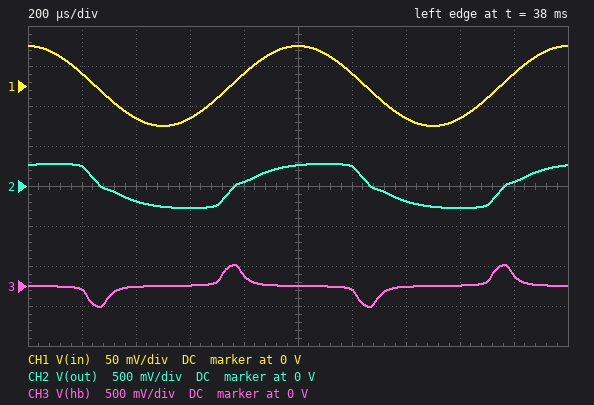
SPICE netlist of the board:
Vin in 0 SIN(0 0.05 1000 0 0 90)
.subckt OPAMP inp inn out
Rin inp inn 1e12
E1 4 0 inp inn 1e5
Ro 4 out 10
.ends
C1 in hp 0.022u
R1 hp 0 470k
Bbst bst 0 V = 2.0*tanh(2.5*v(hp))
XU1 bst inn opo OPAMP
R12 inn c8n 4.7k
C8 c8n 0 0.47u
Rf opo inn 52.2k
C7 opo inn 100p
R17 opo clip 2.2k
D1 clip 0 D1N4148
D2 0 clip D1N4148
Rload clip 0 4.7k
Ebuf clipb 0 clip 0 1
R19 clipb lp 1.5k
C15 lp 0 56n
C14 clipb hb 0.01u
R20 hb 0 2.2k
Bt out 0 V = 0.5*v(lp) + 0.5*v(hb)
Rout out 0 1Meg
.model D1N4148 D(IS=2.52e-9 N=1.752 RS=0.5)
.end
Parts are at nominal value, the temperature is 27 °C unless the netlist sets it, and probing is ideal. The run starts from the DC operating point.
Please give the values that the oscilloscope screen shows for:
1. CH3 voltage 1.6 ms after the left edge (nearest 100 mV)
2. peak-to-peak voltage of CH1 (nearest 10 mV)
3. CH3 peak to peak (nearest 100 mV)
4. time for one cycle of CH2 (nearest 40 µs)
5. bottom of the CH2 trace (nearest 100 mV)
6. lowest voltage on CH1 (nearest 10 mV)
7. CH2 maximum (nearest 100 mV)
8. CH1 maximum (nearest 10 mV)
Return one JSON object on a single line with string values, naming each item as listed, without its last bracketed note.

{"CH3 voltage 1.6 ms after the left edge": "0 V", "peak-to-peak voltage of CH1": "100 mV", "CH3 peak to peak": "500 mV", "time for one cycle of CH2": "1.00 ms", "bottom of the CH2 trace": "-300 mV", "lowest voltage on CH1": "-50 mV", "CH2 maximum": "300 mV", "CH1 maximum": "50 mV"}
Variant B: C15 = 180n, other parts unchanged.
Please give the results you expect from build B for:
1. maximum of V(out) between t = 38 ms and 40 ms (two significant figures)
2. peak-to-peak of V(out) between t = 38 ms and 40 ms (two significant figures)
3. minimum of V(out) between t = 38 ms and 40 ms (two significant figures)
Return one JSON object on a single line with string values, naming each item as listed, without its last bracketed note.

{"maximum of V(out) between t = 38 ms and 40 ms": "170 mV", "peak-to-peak of V(out) between t = 38 ms and 40 ms": "350 mV", "minimum of V(out) between t = 38 ms and 40 ms": "-170 mV"}
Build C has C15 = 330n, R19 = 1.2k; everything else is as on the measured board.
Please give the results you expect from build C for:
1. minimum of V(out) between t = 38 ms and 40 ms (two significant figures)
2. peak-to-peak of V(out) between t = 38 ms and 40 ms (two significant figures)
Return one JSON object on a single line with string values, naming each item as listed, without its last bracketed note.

{"minimum of V(out) between t = 38 ms and 40 ms": "-120 mV", "peak-to-peak of V(out) between t = 38 ms and 40 ms": "250 mV"}
